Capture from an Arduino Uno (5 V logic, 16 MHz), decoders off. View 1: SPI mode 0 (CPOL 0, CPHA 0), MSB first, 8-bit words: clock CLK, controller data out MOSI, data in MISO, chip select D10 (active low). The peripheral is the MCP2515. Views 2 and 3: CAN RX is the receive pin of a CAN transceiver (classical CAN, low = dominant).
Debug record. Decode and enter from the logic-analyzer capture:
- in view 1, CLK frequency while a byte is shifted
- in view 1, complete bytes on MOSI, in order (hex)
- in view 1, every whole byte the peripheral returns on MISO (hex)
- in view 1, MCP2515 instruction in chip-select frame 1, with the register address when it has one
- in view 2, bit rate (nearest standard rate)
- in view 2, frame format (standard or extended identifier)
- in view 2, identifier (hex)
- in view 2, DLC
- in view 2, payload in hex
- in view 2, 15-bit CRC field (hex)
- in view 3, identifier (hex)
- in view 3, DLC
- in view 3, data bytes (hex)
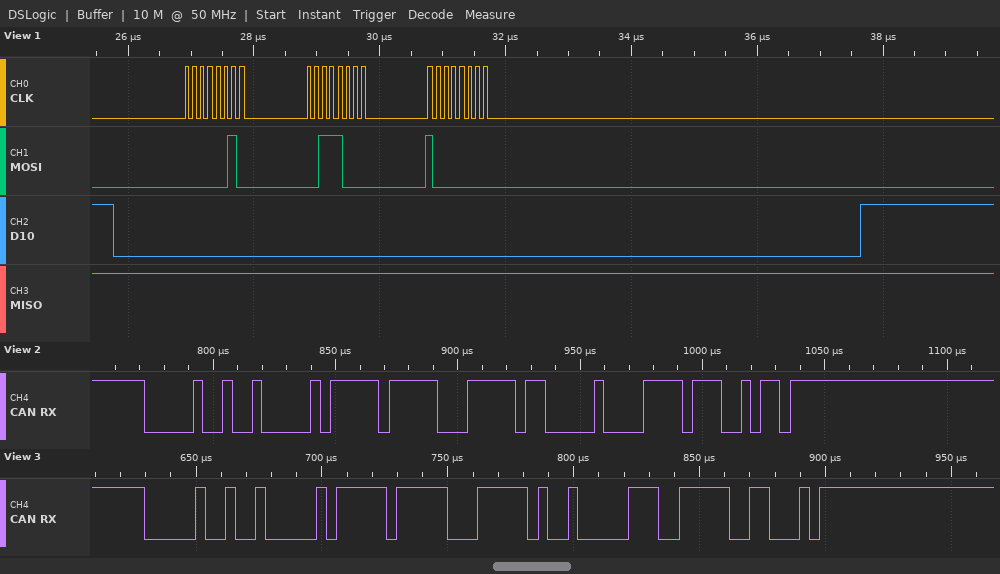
8 MHz
02 38 80
FF FF FF
WRITE 0x38
250 kbit/s
standard
0x012
3
FF 3F 80
0x1EE5
0x012
3
FF 3F 20
